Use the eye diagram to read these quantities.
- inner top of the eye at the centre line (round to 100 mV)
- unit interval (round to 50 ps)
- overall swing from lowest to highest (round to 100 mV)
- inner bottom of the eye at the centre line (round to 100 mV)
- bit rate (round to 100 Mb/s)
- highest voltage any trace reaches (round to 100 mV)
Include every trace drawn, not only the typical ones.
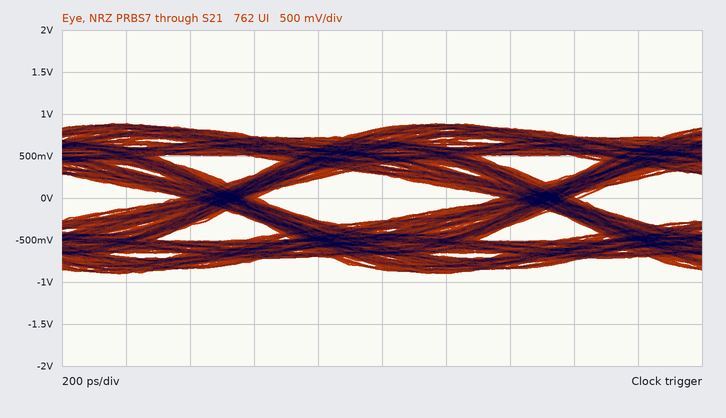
300 mV
1.00 ns
1.8 V
-300 mV
1.0 Gb/s
900 mV
